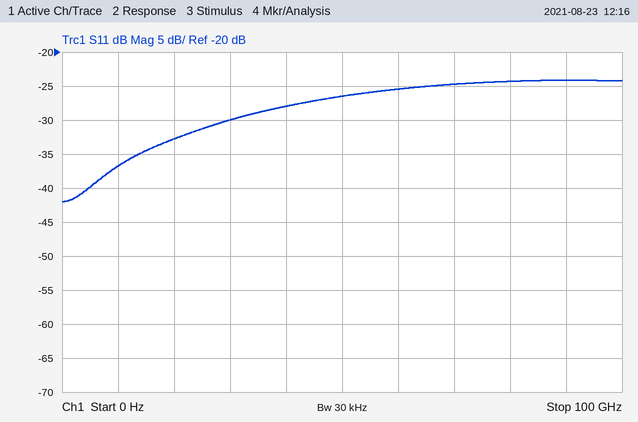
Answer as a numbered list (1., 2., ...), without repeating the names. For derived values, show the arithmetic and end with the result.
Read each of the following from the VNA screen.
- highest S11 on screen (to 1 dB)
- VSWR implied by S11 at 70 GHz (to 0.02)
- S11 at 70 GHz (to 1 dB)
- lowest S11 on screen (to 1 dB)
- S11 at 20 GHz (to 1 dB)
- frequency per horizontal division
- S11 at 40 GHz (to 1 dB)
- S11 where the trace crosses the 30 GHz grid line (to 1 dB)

1. -24 dB
2. |Γ| = 10^(-25/20) = 0.0562; VSWR = (1 + 0.0562)/(1 − 0.0562) ≈ 1.12
3. -25 dB
4. -42 dB
5. -33 dB
6. 10 GHz
7. -28 dB
8. -30 dB
